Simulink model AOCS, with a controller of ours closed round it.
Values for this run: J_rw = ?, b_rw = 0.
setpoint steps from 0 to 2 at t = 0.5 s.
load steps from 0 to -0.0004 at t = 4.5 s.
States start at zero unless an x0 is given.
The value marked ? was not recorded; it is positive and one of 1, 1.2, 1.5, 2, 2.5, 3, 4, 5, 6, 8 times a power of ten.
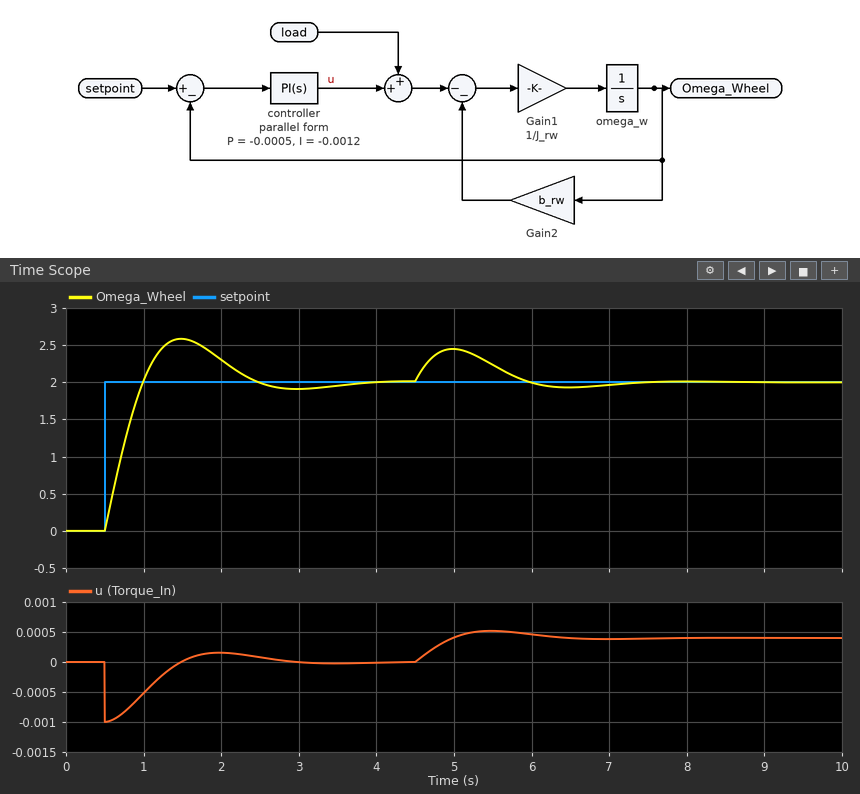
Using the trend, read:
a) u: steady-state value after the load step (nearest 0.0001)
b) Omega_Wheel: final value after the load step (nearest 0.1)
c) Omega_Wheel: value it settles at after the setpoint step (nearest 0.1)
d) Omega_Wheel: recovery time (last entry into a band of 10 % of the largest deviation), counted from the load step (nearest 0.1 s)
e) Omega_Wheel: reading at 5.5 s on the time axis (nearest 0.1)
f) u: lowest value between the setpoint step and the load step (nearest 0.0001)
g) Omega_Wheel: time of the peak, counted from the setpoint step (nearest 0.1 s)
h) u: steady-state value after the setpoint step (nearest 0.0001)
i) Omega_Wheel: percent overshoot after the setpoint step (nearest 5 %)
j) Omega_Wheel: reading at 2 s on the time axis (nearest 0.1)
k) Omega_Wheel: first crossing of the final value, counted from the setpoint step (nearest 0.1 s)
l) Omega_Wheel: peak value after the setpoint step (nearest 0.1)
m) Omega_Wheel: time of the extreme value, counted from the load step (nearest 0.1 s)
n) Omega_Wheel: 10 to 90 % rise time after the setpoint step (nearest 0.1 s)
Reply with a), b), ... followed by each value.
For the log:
a) 0.0004
b) 2.0
c) 2.0
d) 2.4 s
e) 2.2
f) -0.0010
g) 1.0 s
h) 0.0000
i) 30 %
j) 2.3
k) 0.5 s
l) 2.6
m) 0.5 s
n) 0.4 s
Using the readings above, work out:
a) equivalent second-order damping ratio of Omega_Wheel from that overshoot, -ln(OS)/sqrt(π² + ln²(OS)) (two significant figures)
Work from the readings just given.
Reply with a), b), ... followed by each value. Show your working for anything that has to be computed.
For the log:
a) ln(0.3) = -1.204; 1.204 / sqrt(9.870 + 1.450) = 0.36
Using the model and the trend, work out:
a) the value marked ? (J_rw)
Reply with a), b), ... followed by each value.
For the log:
a) 0.0002
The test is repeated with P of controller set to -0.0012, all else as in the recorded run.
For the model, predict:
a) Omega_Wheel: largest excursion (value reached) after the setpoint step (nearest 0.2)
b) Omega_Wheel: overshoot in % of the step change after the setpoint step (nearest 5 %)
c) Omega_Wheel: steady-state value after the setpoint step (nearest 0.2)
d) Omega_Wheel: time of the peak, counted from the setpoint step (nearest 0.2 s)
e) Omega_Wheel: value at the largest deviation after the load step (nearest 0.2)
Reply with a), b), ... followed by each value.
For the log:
a) 2.2
b) 10 %
c) 2.0
d) 0.8 s
e) 2.2
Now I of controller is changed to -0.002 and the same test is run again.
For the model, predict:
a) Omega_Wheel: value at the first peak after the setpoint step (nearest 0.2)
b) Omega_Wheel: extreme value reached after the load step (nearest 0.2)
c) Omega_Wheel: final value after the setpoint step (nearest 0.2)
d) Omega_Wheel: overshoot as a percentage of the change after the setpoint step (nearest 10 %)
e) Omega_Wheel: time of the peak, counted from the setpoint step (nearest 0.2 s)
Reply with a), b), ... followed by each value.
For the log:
a) 2.8
b) 2.4
c) 2.0
d) 40 %
e) 0.8 s
